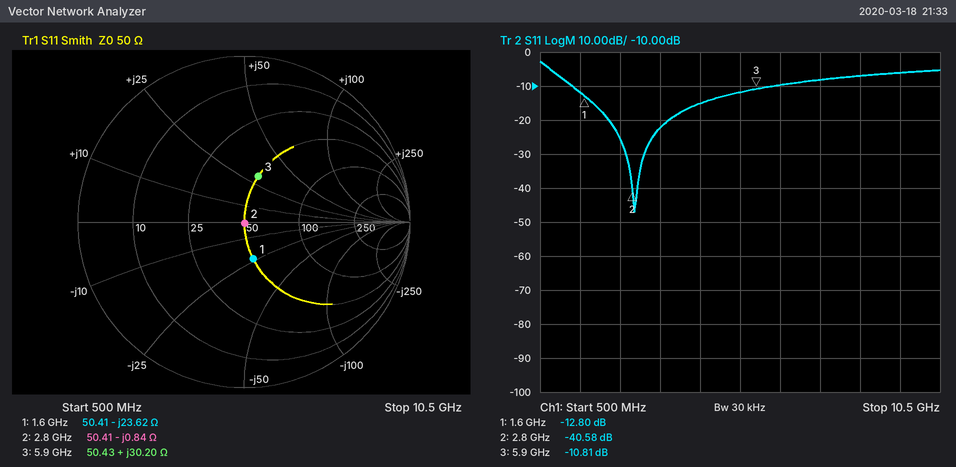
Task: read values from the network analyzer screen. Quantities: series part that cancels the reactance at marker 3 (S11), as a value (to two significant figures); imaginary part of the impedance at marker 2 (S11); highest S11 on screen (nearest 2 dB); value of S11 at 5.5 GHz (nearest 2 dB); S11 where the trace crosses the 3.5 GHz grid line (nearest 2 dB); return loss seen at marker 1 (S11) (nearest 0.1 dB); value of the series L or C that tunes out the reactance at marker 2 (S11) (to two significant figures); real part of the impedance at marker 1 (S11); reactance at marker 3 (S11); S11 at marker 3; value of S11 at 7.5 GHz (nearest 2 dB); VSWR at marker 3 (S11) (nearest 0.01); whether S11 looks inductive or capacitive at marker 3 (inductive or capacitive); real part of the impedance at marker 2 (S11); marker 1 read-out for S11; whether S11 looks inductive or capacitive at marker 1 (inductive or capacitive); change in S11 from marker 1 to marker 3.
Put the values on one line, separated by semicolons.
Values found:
890 fF; -0.84 Ω; -2 dB; -12 dB; -22 dB; 12.8 dB; 48 pH; 50.41 Ω; +30.20 Ω; -10.81 dB; -8 dB; 1.81; inductive; 50.41 Ω; -12.80 dB; capacitive; 1.99 dB
